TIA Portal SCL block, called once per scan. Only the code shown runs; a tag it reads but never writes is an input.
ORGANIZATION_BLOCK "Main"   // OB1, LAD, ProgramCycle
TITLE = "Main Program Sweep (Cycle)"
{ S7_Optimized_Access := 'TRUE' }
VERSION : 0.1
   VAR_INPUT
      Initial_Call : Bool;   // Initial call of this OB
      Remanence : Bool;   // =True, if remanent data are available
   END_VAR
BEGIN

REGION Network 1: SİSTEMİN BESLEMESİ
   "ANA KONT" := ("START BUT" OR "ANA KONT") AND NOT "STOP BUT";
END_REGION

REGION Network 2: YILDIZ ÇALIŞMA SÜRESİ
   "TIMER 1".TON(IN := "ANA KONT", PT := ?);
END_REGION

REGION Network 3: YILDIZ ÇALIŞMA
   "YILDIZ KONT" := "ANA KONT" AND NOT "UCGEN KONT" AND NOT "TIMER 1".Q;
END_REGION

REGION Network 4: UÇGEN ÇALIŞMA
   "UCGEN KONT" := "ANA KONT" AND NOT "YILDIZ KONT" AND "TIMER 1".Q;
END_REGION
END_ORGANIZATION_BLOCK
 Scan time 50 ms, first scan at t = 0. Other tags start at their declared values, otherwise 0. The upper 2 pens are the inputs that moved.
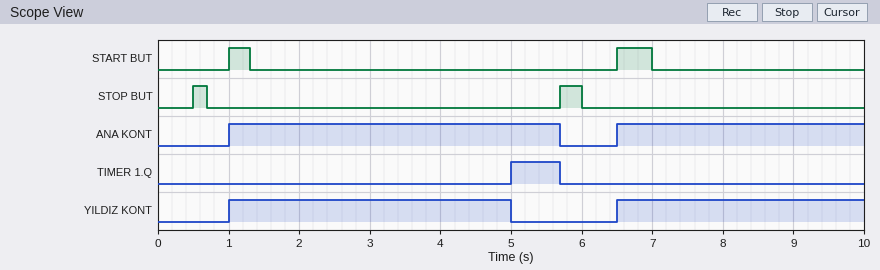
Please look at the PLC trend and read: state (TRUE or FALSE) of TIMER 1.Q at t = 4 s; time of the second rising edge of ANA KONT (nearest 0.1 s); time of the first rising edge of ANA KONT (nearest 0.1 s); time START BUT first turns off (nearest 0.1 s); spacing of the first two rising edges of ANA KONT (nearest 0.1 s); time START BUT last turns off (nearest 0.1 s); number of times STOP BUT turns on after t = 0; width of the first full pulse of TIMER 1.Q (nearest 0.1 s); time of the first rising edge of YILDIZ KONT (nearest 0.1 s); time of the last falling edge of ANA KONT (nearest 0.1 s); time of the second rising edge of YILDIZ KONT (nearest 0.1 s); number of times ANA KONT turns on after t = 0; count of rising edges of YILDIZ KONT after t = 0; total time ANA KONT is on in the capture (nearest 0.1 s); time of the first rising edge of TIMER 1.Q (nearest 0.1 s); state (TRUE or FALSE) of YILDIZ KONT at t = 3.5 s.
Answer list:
FALSE
6.5 s
1.0 s
1.3 s
5.5 s
7.0 s
2
0.7 s
1.0 s
5.7 s
6.5 s
2
2
8.2 s
5.0 s
TRUE
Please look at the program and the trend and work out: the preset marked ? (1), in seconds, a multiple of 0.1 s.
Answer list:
4.0 s
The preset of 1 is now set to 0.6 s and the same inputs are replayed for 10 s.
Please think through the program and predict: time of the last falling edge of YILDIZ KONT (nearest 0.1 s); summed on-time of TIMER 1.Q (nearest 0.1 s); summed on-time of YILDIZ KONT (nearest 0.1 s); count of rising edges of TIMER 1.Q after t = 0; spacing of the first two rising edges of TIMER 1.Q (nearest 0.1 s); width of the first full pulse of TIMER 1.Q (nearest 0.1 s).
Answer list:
7.1 s
7.0 s
1.2 s
2
5.5 s
4.1 s
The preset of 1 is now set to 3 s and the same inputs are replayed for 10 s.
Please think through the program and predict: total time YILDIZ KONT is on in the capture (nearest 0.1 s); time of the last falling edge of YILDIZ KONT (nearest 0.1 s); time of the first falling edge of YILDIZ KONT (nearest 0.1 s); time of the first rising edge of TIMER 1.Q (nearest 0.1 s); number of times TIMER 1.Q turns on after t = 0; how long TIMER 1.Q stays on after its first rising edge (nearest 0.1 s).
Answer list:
6.0 s
9.5 s
4.0 s
4.0 s
2
1.7 s
